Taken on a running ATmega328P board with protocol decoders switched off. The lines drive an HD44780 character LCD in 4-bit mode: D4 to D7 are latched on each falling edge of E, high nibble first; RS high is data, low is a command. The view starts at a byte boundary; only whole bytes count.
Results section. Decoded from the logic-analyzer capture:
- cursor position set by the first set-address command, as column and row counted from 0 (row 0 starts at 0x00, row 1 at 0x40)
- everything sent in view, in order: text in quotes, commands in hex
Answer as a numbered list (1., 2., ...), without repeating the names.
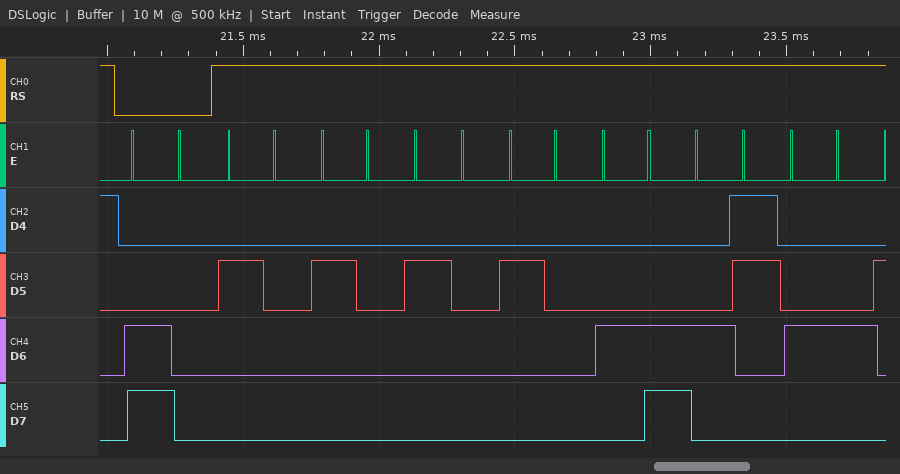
1. column 0, row 1
2. 0xC0 "    LCD"
